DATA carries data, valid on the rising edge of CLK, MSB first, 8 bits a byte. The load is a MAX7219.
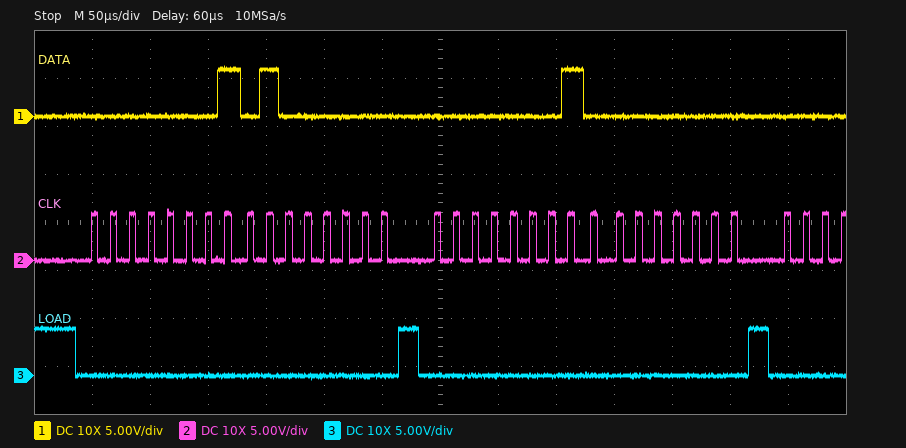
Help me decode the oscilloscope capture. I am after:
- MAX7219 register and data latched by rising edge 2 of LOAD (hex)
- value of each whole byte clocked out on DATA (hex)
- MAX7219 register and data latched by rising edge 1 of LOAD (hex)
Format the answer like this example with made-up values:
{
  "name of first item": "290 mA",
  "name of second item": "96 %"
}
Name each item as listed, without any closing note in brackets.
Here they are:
{
  "MAX7219 register and data latched by rising edge 2 of LOAD": "register 0x1, data 0x00",
  "value of each whole byte clocked out on DATA": "01 40 01 00",
  "MAX7219 register and data latched by rising edge 1 of LOAD": "register 0x1, data 0x40"
}
